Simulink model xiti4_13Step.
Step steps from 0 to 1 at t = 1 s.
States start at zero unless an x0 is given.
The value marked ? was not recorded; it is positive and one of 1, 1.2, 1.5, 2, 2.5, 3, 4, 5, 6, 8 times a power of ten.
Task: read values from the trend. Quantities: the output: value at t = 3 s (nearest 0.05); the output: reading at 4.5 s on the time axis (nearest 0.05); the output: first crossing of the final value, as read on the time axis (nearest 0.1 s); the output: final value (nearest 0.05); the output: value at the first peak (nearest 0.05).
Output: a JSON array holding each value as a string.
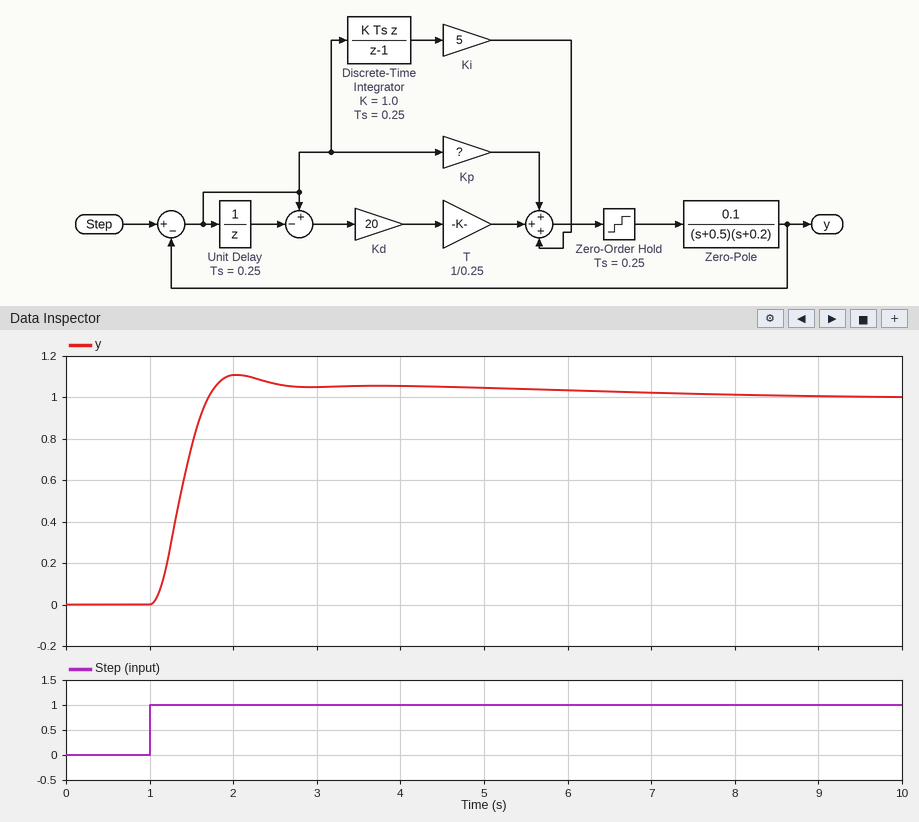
["1.05", "1.05", "1.7 s", "1.00", "1.10"]
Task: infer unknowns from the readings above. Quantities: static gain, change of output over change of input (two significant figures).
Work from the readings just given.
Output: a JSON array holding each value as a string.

["1.0"]
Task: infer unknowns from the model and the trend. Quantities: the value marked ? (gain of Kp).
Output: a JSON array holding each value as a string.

["15"]
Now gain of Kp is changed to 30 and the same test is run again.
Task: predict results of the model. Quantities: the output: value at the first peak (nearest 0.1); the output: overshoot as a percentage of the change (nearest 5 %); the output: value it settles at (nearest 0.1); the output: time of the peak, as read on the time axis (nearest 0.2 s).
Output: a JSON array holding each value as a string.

["1.3", "30 %", "1.0", "2.0 s"]
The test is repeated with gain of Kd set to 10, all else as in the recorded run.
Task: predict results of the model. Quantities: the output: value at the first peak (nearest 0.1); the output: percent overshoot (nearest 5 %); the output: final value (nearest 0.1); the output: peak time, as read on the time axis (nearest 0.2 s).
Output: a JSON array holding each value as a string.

["1.3", "25 %", "1.0", "3.0 s"]
